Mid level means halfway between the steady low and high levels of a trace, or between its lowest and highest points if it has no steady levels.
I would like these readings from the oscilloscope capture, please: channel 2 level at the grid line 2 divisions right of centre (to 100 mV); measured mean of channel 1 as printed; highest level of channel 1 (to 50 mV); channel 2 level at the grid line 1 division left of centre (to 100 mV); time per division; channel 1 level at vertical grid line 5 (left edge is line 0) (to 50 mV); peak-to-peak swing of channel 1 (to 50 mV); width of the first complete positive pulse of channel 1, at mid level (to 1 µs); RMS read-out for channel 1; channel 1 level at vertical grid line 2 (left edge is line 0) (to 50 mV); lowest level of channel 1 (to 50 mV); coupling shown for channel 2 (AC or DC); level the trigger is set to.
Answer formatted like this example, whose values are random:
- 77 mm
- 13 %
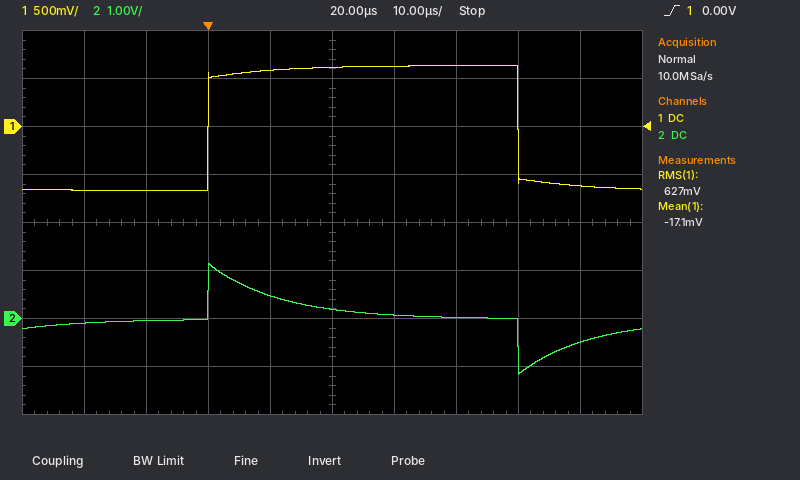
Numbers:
- 0.0 V
- -17.1 mV
- 650 mV
- 500 mV
- 10 µs
- 600 mV
- 1.30 V
- 50 µs
- 627 mV
- -650 mV
- -650 mV
- DC
- 0.00 V
